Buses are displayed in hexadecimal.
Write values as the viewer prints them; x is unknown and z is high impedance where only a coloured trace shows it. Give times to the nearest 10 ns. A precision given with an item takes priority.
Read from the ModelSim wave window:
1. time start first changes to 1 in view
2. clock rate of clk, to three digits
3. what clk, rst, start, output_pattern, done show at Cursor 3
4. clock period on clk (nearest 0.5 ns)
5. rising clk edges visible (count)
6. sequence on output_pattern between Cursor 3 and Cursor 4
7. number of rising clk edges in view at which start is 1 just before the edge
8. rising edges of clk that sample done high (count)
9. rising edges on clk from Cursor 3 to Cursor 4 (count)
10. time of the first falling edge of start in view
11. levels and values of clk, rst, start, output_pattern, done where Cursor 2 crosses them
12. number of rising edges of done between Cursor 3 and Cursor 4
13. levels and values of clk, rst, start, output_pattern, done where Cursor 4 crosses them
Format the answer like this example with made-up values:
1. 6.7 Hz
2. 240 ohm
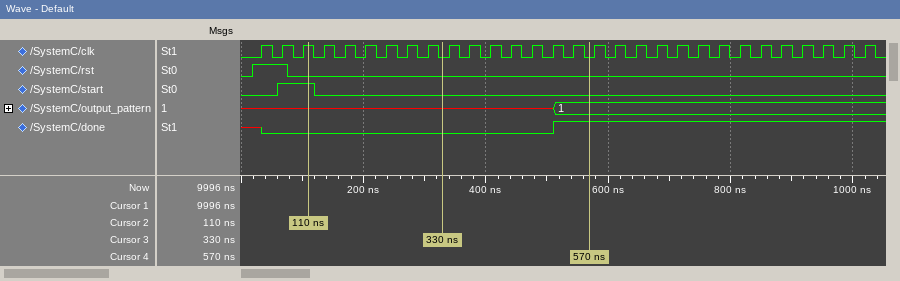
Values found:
1. 60 ns
2. 29.4 MHz
3. clk=0, rst=0, start=0, output_pattern=x, done=0
4. 34 ns
5. 30
6. x, 1
7. 2
8. 15
9. 7
10. 120 ns
11. clk=1, rst=0, start=1, output_pattern=x, done=0
12. 1
13. clk=0, rst=0, start=0, output_pattern=1, done=1
